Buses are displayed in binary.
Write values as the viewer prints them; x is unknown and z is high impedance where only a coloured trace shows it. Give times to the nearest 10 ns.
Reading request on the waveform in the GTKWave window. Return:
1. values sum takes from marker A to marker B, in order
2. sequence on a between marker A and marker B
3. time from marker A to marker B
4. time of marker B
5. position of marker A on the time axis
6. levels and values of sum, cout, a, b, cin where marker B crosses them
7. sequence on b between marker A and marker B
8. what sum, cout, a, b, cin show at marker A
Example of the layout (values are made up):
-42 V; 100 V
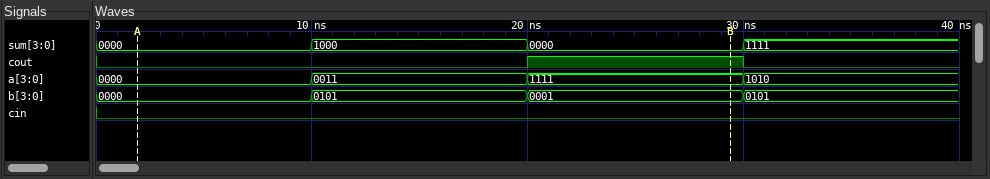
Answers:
0000, 1000, 0000; 0000, 0011, 1111; 30 ns; 30 ns; 0 ns; sum=0000, cout=1, a=1111, b=0001, cin=0; 0000, 0101, 0001; sum=0000, cout=0, a=0000, b=0000, cin=0
